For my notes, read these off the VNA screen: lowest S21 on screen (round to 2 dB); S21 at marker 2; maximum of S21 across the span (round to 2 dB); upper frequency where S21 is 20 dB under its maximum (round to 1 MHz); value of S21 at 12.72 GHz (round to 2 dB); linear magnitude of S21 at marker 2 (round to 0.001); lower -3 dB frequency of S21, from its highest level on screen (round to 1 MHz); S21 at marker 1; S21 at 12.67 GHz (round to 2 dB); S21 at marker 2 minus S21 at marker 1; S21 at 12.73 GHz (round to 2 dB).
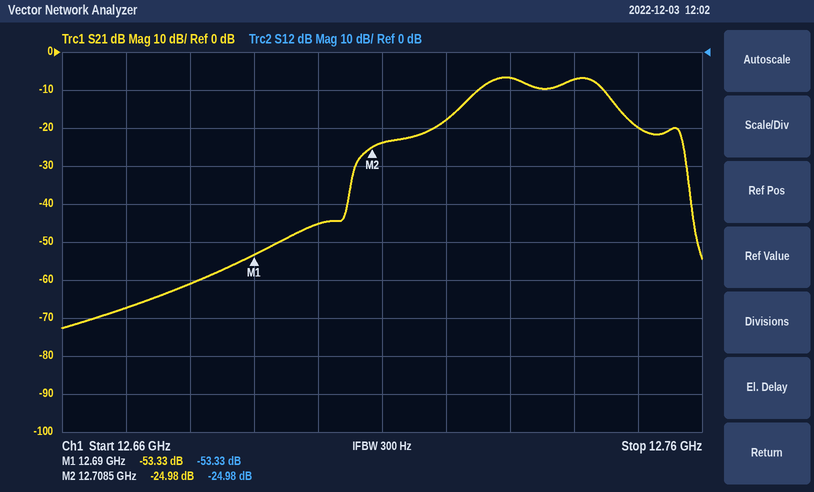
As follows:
-72 dB
-24.98 dB
-6 dB
12.757 GHz
-18 dB
0.056
12.725 GHz
-53.33 dB
-68 dB
28.35 dB
-6 dB
